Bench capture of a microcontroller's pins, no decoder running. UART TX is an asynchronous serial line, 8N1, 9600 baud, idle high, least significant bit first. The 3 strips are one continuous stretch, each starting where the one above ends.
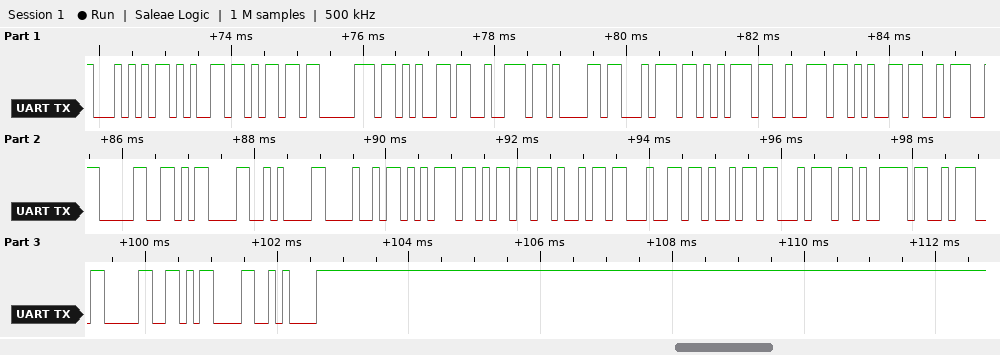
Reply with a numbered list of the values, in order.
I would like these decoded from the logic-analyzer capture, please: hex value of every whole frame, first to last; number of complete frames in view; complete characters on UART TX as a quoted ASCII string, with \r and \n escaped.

1. 54 65 6D 70 65 72 61 74 75 72 65 3A 30 0D 0A 48 75 6D 69 64 69 74 79 3A 30 0D 0A
2. 27
3. "Temperature:0\r\nHumidity:0\r\n"
